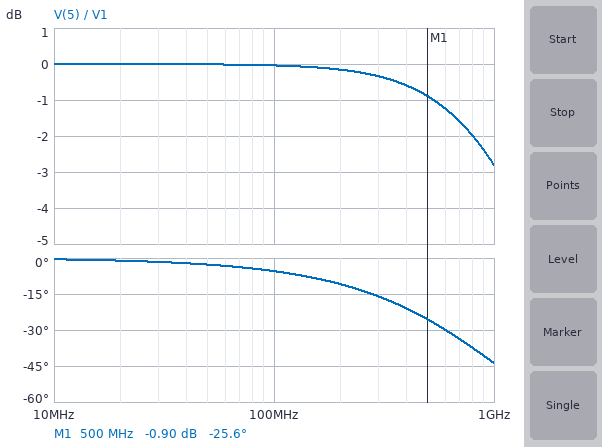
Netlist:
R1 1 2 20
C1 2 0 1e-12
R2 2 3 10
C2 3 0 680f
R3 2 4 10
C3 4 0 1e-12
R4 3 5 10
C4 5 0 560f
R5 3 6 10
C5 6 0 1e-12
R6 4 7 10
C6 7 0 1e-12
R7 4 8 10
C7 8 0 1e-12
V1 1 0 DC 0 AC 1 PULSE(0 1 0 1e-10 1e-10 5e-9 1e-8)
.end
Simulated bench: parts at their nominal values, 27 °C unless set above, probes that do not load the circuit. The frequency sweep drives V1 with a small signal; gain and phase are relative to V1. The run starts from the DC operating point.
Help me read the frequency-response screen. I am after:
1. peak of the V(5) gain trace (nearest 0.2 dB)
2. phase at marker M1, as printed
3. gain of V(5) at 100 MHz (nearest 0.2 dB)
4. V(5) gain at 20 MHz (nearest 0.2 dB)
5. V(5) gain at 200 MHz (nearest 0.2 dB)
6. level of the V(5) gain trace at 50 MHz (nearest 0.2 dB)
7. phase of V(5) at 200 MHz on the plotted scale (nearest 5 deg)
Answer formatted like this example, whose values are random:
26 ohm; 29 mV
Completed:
0 dB; -25.6 deg; 0 dB; 0 dB; -0.2 dB; 0 dB; -10 deg
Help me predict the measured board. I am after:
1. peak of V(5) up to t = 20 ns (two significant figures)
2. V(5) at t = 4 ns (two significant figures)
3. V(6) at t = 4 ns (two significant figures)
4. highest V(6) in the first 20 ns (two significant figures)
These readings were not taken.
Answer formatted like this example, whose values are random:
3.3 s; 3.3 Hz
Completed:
1.0 V; 1.0 V; 1.0 V; 1.0 V
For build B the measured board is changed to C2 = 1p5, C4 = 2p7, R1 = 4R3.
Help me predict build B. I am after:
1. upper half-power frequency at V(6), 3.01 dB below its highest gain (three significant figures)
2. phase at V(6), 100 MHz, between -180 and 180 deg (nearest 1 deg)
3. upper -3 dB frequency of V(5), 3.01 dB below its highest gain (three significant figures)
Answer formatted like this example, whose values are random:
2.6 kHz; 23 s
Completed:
1.59 GHz; -4 deg; 1.50 GHz
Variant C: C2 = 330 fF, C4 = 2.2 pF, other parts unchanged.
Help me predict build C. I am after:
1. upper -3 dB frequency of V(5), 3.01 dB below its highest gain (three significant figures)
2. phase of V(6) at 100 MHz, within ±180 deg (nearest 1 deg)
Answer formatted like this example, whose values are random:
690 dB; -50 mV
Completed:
817 MHz; -7 deg
